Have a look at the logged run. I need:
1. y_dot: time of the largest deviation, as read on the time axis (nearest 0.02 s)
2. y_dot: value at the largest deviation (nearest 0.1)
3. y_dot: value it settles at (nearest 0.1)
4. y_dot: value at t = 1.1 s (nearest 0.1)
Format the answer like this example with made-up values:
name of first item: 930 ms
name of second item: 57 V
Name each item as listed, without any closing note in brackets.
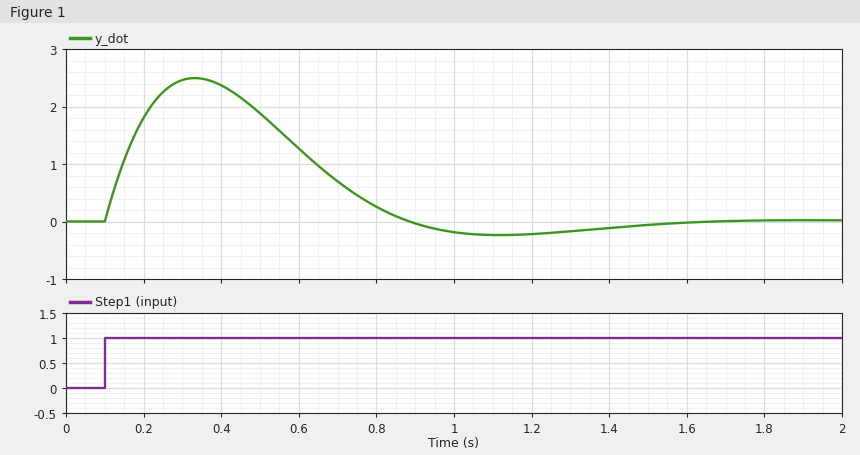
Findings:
y_dot: time of the largest deviation, as read on the time axis: 0.34 s
y_dot: value at the largest deviation: 2.5
y_dot: value it settles at: 0.0
y_dot: value at t = 1.1 s: -0.2
